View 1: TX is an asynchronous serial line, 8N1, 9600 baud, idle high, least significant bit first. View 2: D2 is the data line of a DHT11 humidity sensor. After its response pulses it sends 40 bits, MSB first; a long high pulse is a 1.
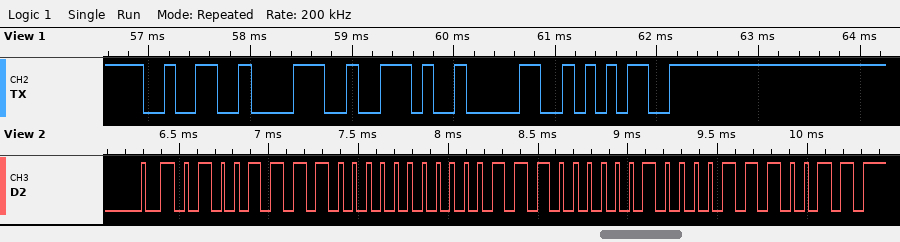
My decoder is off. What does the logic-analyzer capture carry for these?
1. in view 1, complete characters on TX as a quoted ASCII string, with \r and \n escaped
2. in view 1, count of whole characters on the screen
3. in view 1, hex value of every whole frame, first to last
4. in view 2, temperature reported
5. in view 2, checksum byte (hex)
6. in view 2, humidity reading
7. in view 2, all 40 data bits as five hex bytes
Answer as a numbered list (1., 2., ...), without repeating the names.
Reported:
1. "28.05"
2. 5
3. 0x32 0x38 0x2E 0x30 0x35
4. 28.8 °C
5. 0x73
6. 79 %
7. 4F 00 1C 08 73
